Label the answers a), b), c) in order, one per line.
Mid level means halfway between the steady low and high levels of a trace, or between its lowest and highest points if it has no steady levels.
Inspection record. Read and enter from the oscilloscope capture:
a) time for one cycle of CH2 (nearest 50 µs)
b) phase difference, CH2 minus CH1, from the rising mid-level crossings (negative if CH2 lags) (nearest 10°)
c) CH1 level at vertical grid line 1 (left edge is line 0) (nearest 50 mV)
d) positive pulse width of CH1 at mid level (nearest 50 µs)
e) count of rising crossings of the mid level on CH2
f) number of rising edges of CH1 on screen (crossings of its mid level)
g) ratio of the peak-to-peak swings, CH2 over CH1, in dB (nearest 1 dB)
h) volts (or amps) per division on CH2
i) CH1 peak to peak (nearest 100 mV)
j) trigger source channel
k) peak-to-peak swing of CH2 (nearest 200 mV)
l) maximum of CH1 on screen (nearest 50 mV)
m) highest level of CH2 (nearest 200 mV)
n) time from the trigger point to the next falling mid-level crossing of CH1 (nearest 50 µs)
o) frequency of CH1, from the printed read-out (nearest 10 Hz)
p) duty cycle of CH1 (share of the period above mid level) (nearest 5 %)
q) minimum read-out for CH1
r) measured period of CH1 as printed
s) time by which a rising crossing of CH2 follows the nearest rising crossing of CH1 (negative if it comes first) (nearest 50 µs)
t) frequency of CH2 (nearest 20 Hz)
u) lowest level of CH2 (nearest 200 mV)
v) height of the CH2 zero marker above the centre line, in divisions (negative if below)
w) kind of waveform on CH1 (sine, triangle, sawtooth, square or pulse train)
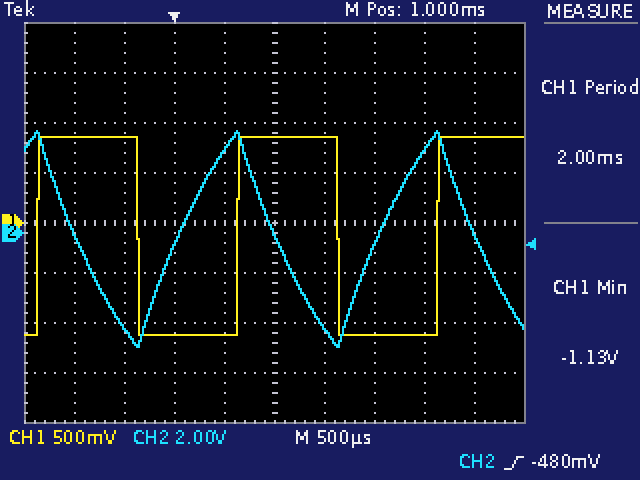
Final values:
a) 2.00 ms
b) +110°
c) 850 mV
d) 1.00 ms
e) 2
f) 3
g) 13 dB
h) 2 V
i) 2.00 V
j) CH2
k) 8.6 V
l) 850 mV
m) 4.0 V
n) 1.65 ms
o) 500 Hz
p) 50 %
q) -1.13 V
r) 2.00 ms
s) -600 µs
t) 500 Hz
u) -4.6 V
v) -0.2 div
w) square
